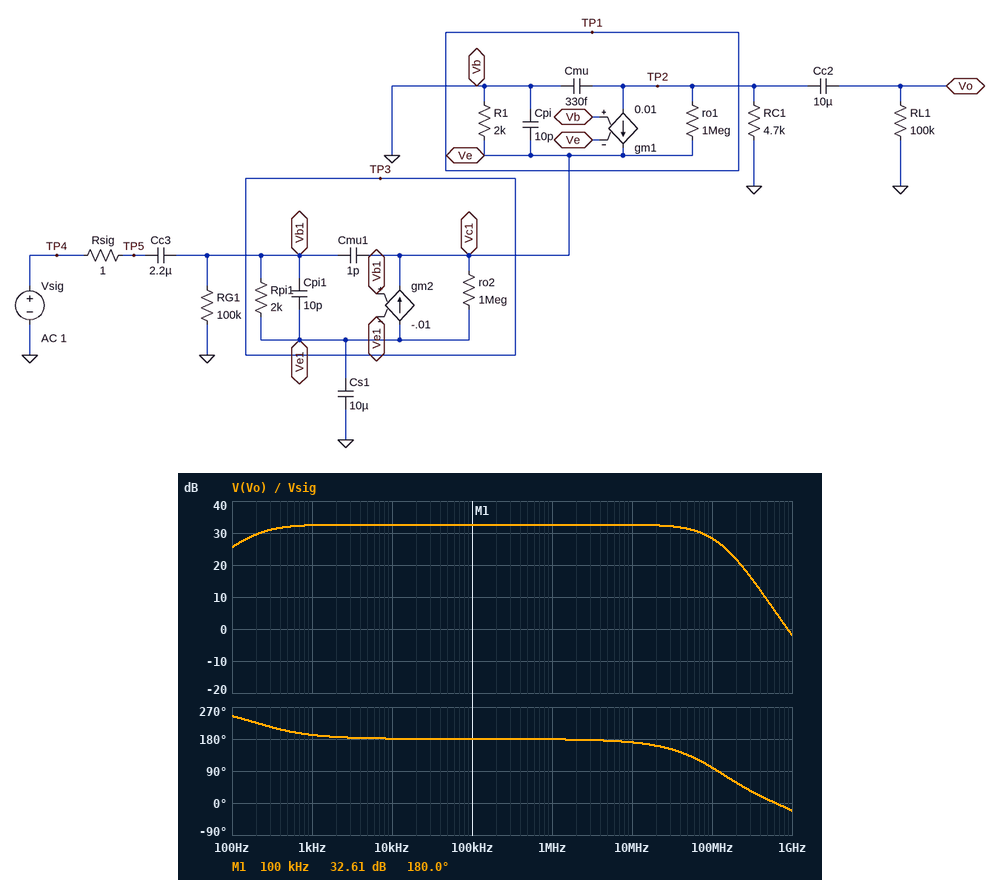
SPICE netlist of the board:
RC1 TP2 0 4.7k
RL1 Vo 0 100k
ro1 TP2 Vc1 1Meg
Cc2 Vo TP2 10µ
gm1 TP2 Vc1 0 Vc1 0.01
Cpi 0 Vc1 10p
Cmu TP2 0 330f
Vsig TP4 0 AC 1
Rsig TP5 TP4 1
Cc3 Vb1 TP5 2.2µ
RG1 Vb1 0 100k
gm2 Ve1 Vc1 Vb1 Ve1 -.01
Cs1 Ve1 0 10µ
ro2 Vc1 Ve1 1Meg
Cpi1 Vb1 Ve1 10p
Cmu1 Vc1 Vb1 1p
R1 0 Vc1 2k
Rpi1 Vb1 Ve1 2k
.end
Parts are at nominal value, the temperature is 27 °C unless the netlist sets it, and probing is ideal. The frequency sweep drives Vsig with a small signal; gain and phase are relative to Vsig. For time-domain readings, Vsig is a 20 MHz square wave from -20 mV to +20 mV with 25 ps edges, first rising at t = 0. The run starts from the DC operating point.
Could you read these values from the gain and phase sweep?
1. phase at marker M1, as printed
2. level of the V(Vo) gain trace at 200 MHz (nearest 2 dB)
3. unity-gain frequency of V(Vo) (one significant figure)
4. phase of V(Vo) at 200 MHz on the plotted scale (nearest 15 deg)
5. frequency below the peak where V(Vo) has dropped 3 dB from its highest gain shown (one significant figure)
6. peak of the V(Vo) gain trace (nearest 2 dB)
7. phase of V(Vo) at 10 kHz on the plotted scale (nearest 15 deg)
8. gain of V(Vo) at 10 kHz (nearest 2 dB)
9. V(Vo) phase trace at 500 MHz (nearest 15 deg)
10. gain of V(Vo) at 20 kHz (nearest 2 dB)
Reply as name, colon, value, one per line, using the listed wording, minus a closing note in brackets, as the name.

phase at marker M1, as printed: 180.0 deg
level of the V(Vo) gain trace at 200 MHz: 22 dB
unity-gain frequency of V(Vo): 900 MHz
phase of V(Vo) at 200 MHz on the plotted scale: 60 deg
frequency below the peak where V(Vo) has dropped 3 dB from its highest gain shown: 200 Hz
peak of the V(Vo) gain trace: 32 dB
phase of V(Vo) at 10 kHz on the plotted scale: 180 deg
gain of V(Vo) at 10 kHz: 32 dB
V(Vo) phase trace at 500 MHz: 15 deg
gain of V(Vo) at 20 kHz: 32 dB
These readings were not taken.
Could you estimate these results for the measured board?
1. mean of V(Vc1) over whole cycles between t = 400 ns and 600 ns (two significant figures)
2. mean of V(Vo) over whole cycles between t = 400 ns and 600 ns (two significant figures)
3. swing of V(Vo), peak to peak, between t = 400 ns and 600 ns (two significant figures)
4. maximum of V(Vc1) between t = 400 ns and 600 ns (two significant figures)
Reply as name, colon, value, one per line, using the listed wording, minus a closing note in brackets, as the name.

mean of V(Vc1) over whole cycles between t = 400 ns and 600 ns: -19 mV
mean of V(Vo) over whole cycles between t = 400 ns and 600 ns: -850 mV
swing of V(Vo), peak to peak, between t = 400 ns and 600 ns: 1.7 V
maximum of V(Vc1) between t = 400 ns and 600 ns: 2.6 mV
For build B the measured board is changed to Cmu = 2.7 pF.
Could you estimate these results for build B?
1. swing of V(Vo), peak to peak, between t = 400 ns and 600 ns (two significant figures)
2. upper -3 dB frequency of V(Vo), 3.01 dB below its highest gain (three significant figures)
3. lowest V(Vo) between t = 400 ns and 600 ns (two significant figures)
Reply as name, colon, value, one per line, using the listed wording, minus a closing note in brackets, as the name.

swing of V(Vo), peak to peak, between t = 400 ns and 600 ns: 1.3 V
upper -3 dB frequency of V(Vo), 3.01 dB below its highest gain: 13.0 MHz
lowest V(Vo) between t = 400 ns and 600 ns: -1.5 V
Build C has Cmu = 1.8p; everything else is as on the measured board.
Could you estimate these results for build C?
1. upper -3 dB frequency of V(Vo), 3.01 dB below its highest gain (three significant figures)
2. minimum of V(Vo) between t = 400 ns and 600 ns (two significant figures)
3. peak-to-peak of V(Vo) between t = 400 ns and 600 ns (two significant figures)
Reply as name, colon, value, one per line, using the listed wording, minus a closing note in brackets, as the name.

upper -3 dB frequency of V(Vo), 3.01 dB below its highest gain: 19.4 MHz
minimum of V(Vo) between t = 400 ns and 600 ns: -1.6 V
peak-to-peak of V(Vo) between t = 400 ns and 600 ns: 1.5 V
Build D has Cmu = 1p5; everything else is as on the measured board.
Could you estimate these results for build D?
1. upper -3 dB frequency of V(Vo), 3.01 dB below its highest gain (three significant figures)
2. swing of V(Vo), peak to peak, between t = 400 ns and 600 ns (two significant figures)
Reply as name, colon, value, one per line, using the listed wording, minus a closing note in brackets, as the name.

upper -3 dB frequency of V(Vo), 3.01 dB below its highest gain: 23.1 MHz
swing of V(Vo), peak to peak, between t = 400 ns and 600 ns: 1.6 V
